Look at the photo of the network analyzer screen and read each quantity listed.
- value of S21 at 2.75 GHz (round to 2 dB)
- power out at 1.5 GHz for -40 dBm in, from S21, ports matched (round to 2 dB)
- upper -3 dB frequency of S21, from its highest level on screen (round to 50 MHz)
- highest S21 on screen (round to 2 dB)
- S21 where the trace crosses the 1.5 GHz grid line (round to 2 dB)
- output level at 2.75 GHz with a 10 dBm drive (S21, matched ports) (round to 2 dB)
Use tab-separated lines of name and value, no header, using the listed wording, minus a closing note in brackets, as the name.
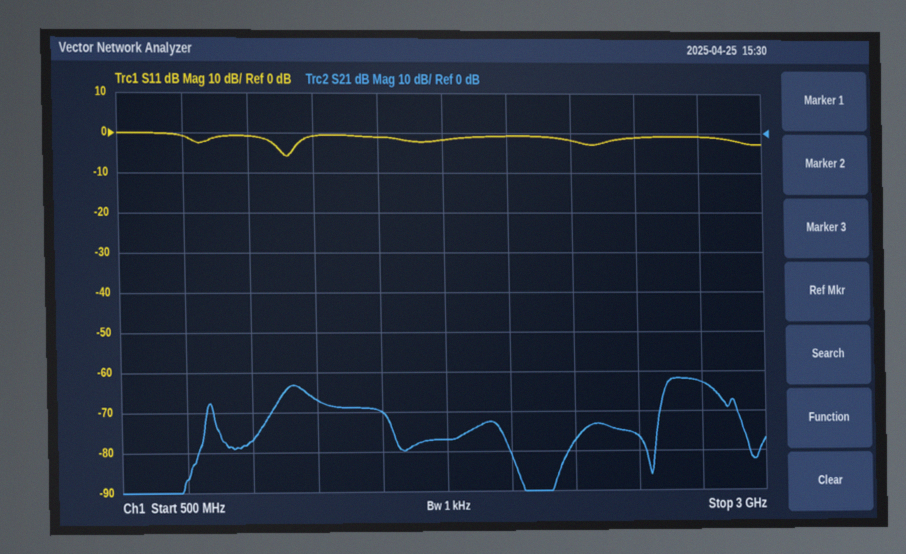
value of S21 at 2.75 GHz	-62 dB
power out at 1.5 GHz for -40 dBm in, from S21, ports matched	-110 dBm
upper -3 dB frequency of S21, from its highest level on screen	2.80 GHz
highest S21 on screen	-62 dB
S21 where the trace crosses the 1.5 GHz grid line	-70 dB
output level at 2.75 GHz with a 10 dBm drive (S21, matched ports)	-52 dBm
